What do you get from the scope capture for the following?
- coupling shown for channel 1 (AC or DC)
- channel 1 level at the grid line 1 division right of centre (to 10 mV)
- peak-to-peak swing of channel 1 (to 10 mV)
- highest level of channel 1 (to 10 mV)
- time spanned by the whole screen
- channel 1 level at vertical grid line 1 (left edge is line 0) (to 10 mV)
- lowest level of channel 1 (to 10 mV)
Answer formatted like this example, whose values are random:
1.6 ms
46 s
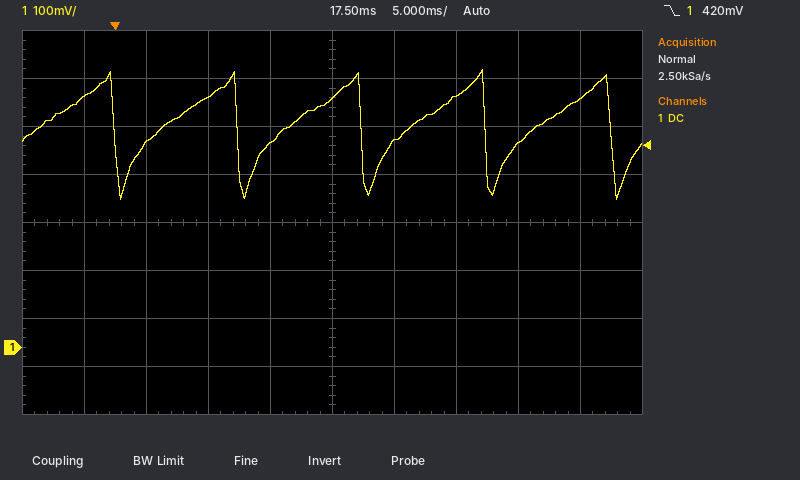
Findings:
DC
430 mV
270 mV
580 mV
50 ms
520 mV
310 mV
